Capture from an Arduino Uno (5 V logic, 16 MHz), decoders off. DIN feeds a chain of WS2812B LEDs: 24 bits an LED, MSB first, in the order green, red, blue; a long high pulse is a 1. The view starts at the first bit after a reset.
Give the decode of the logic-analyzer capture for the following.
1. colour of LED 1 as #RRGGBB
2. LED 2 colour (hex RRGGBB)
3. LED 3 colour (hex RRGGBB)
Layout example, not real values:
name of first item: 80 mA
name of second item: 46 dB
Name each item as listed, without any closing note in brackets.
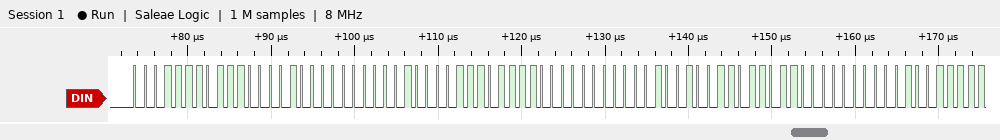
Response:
colour of LED 1 as #RRGGBB: #E11E00
LED 2 colour: #DE2100
LED 3 colour: #DB2400
